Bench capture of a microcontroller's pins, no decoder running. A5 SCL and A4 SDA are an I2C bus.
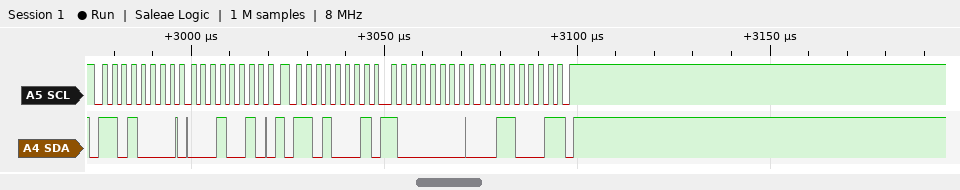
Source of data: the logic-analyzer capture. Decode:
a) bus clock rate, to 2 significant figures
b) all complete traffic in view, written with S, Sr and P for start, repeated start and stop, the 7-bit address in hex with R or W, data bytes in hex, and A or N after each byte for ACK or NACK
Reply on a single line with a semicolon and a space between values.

400 kHz; S 68W A 12 A Sr 68R A 80 A 31 N P
